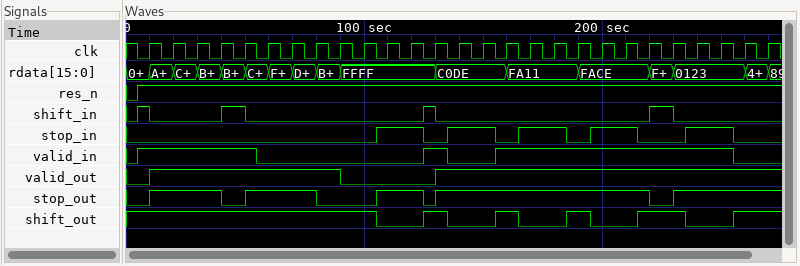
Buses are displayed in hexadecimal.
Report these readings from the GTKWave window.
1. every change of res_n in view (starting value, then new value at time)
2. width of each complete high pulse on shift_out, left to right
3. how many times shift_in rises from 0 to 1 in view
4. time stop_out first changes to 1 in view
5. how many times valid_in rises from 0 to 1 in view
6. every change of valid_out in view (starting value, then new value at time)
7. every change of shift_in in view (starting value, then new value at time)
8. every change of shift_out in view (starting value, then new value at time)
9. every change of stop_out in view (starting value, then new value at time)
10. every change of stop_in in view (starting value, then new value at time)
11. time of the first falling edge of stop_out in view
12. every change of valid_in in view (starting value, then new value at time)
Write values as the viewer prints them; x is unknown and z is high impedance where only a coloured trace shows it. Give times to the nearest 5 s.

0, 1 at 5 s
10 s, 10 s, 10 s, 20 s
4
10 s
3
0, 1 at 10 s, 0 at 90 s, 1 at 130 s
0, 1 at 5 s, 0 at 10 s, 1 at 40 s, 0 at 50 s, 1 at 125 s, 0 at 130 s, 1 at 220 s, 0 at 230 s
1, 0 at 105 s, 1 at 125 s, 0 at 135 s, 1 at 155 s, 0 at 165 s, 1 at 185 s, 0 at 195 s, 1 at 215 s, 0 at 235 s, 1 at 255 s
0, 1 at 10 s, 0 at 40 s, 1 at 50 s, 0 at 80 s, 1 at 105 s, 0 at 125 s, 1 at 130 s, 0 at 220 s, 1 at 230 s
0, 1 at 105 s, 0 at 125 s, 1 at 135 s, 0 at 155 s, 1 at 165 s, 0 at 185 s, 1 at 195 s, 0 at 215 s, 1 at 235 s, 0 at 255 s
40 s
0, 1 at 5 s, 0 at 55 s, 1 at 125 s, 0 at 135 s, 1 at 155 s, 0 at 255 s
